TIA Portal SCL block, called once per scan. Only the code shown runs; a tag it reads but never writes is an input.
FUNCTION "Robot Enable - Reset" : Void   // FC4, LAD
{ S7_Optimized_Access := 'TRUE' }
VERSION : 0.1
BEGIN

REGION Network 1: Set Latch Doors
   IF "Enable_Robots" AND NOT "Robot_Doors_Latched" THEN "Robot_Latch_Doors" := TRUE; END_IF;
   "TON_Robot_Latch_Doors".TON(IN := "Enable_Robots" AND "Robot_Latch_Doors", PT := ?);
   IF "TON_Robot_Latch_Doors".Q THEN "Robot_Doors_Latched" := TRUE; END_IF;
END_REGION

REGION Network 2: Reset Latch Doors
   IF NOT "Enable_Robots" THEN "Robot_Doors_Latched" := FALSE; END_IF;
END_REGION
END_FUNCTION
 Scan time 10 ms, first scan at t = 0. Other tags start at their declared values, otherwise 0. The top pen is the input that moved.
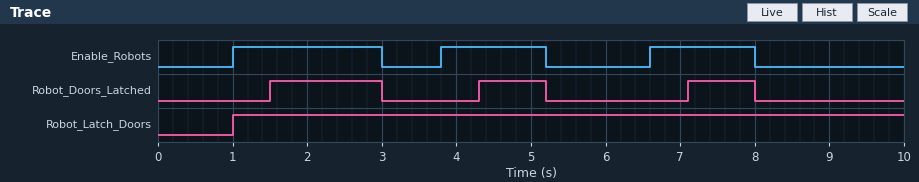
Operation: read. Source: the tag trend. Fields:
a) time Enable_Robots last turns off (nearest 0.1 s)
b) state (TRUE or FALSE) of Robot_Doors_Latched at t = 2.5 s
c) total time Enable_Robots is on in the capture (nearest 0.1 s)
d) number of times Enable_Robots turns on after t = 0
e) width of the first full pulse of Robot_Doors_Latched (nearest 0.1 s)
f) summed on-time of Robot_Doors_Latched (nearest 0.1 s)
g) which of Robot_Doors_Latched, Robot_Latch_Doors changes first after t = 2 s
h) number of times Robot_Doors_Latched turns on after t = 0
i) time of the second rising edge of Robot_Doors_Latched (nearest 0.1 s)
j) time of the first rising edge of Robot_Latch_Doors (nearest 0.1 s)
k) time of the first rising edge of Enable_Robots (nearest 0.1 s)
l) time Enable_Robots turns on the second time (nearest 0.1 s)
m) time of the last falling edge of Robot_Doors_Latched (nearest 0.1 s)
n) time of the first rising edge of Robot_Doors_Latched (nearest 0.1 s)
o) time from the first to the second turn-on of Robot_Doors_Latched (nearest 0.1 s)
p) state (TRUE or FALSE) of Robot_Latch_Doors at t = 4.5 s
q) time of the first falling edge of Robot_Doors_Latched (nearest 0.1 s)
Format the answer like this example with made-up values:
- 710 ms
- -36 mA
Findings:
- 8.0 s
- TRUE
- 4.8 s
- 3
- 1.5 s
- 3.3 s
- Robot_Doors_Latched
- 3
- 4.3 s
- 1.0 s
- 1.0 s
- 3.8 s
- 8.0 s
- 1.5 s
- 2.8 s
- TRUE
- 3.0 s
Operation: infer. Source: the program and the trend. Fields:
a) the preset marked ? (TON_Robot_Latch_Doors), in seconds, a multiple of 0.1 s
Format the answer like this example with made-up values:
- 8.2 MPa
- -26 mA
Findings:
- 0.5 s
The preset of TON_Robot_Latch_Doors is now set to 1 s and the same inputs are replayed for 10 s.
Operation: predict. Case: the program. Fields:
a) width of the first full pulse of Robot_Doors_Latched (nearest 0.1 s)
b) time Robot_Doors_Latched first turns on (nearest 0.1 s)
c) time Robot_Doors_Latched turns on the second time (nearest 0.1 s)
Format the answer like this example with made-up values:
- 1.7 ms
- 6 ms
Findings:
- 1.0 s
- 2.0 s
- 4.8 s
